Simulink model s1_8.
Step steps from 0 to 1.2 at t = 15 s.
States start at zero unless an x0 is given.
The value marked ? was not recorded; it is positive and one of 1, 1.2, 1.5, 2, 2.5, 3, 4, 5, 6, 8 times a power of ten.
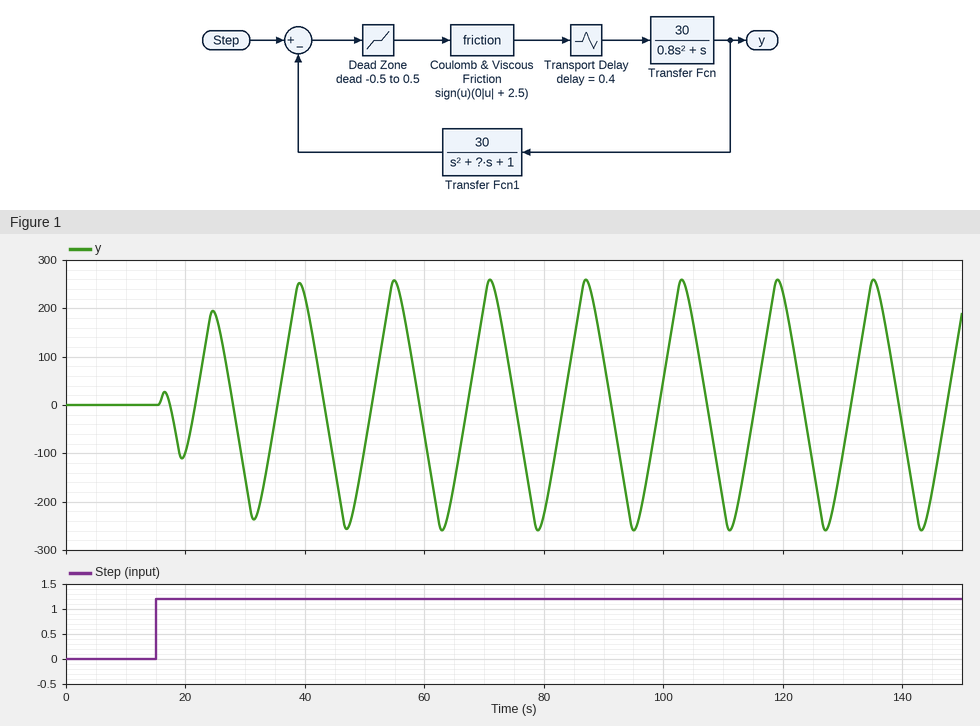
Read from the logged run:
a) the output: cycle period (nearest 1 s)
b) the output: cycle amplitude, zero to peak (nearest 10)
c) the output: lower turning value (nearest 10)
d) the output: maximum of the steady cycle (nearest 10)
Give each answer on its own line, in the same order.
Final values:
16 s
260
-260
260
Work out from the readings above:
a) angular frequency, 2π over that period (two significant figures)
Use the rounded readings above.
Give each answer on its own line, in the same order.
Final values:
0.39 rad/s
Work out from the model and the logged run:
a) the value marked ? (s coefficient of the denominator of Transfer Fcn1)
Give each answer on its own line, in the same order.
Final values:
4
